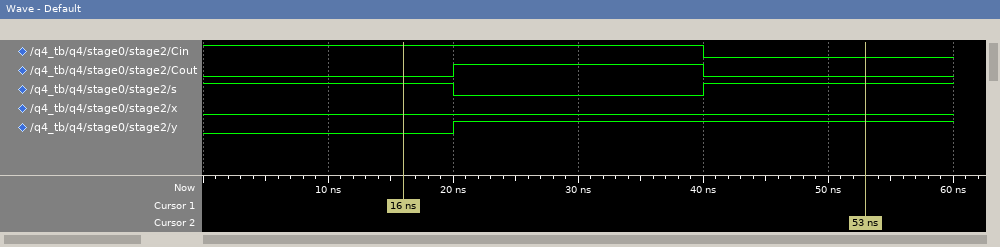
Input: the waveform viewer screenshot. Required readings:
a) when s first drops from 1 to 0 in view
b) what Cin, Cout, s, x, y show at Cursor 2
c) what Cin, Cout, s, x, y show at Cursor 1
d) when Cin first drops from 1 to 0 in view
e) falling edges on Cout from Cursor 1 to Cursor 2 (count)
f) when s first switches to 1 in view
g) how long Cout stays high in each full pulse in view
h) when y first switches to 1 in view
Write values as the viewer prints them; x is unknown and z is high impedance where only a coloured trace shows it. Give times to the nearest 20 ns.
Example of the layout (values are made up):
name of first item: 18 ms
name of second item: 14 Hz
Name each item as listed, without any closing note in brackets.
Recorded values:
when s first drops from 1 to 0 in view: 20 ns
what Cin, Cout, s, x, y show at Cursor 2: Cin=0, Cout=0, s=1, x=0, y=1
what Cin, Cout, s, x, y show at Cursor 1: Cin=1, Cout=0, s=1, x=0, y=0
when Cin first drops from 1 to 0 in view: 40 ns
falling edges on Cout from Cursor 1 to Cursor 2: 1
when s first switches to 1 in view: 40 ns
how long Cout stays high in each full pulse in view: 20 ns
when y first switches to 1 in view: 20 ns
